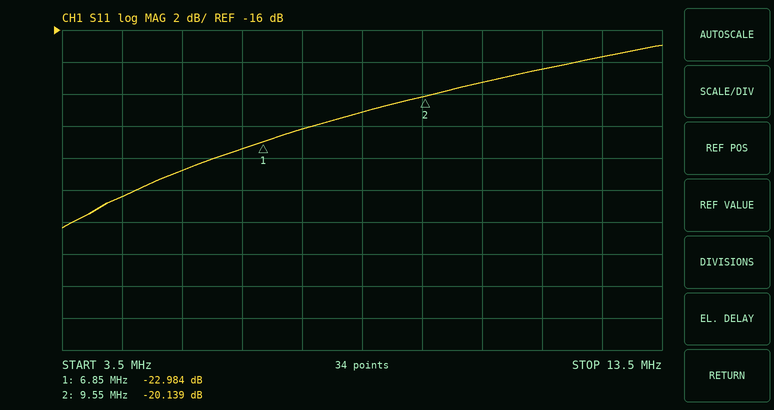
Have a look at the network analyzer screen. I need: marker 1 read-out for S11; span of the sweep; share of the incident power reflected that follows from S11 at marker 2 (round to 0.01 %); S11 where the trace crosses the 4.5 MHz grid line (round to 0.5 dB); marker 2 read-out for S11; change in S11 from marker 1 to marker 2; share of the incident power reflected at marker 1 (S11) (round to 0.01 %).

-22.984 dB
10 MHz
0.97 %
-26.5 dB
-20.139 dB
2.845 dB
0.50 %
